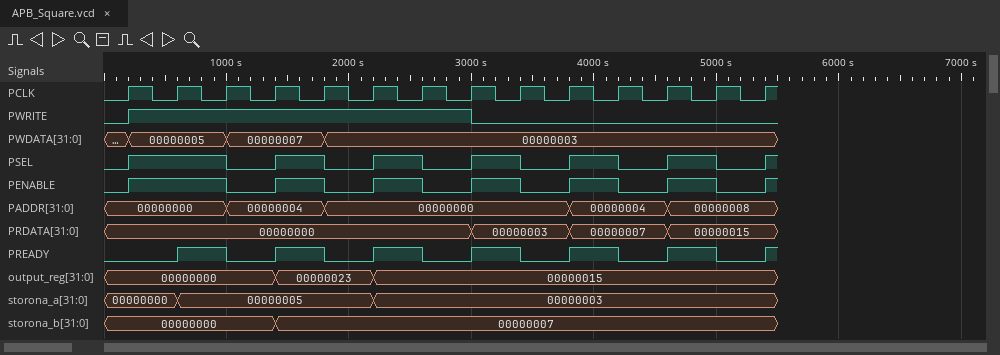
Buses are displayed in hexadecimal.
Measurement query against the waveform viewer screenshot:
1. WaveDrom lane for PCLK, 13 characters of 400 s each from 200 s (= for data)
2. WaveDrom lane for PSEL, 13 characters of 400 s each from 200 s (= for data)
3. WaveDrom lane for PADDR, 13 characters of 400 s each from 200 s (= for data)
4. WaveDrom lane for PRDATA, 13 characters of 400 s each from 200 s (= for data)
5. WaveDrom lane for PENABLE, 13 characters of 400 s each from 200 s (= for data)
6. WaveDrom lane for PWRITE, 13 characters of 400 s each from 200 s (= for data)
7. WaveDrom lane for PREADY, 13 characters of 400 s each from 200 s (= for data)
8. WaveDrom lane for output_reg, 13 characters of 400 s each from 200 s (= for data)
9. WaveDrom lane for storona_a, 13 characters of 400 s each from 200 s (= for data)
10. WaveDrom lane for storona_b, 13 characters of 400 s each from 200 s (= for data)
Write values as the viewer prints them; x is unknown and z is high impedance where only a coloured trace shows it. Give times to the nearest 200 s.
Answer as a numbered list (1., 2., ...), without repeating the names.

1. {name: 'PCLK', wave: 'p............'}
2. {name: 'PSEL', wave: '1.01010101010'}
3. {name: 'PADDR', wave: '=.=.=....=.=.', data: '00000000 00000004 00000000 00000004 00000008'}
4. {name: 'PRDATA', wave: '=......=.=.=.', data: '00000000 00000003 00000007 00000015'}
5. {name: 'PENABLE', wave: '1.01010101010'}
6. {name: 'PWRITE', wave: '1......0.....'}
7. {name: 'PREADY', wave: '0101010101010'}
8. {name: 'output_reg', wave: '=..=.=.......', data: '00000000 00000023 00000015'}
9. {name: 'storona_a', wave: '==...=.......', data: '00000000 00000005 00000003'}
10. {name: 'storona_b', wave: '=..=.........', data: '00000000 00000007'}
